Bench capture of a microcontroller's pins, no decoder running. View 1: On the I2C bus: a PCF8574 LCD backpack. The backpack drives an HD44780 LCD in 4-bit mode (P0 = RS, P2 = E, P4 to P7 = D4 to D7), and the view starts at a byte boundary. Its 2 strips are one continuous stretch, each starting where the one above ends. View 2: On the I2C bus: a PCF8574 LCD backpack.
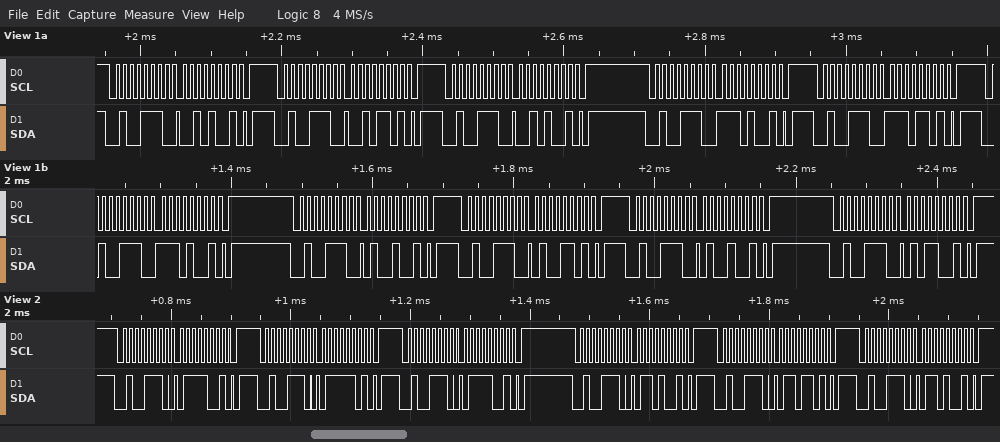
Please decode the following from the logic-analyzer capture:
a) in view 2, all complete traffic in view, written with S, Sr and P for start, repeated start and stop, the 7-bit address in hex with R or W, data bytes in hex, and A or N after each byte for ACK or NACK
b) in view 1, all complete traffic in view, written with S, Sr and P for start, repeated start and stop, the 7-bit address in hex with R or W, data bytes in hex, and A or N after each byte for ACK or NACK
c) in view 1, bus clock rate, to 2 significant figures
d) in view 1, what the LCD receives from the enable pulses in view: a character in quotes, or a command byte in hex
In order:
S 27W A 79 A P S 27W A 7D A P S 27W A 79 A P S 27W A 69 A P S 27W A 6D A P S 27W A 69 A P
S 27W A 29 A P S 27W A 2D A P S 27W A 29 A P S 27W A E9 A P S 27W A ED A P S 27W A E9 A P S 27W A 49 A P S 27W A 4D A P S 27W A 49 A P S 27W A 59 A P
100 kHz
'.'
